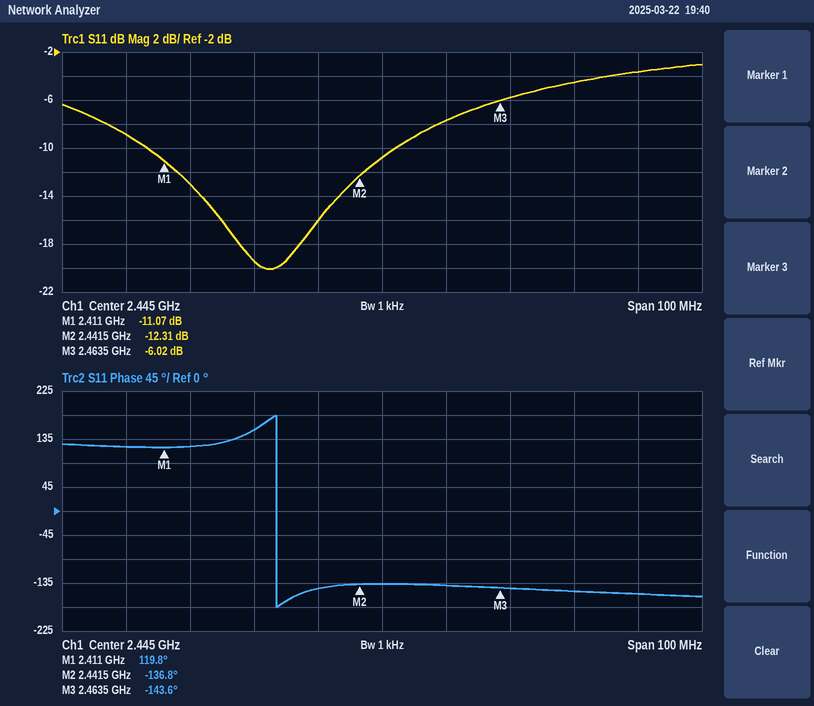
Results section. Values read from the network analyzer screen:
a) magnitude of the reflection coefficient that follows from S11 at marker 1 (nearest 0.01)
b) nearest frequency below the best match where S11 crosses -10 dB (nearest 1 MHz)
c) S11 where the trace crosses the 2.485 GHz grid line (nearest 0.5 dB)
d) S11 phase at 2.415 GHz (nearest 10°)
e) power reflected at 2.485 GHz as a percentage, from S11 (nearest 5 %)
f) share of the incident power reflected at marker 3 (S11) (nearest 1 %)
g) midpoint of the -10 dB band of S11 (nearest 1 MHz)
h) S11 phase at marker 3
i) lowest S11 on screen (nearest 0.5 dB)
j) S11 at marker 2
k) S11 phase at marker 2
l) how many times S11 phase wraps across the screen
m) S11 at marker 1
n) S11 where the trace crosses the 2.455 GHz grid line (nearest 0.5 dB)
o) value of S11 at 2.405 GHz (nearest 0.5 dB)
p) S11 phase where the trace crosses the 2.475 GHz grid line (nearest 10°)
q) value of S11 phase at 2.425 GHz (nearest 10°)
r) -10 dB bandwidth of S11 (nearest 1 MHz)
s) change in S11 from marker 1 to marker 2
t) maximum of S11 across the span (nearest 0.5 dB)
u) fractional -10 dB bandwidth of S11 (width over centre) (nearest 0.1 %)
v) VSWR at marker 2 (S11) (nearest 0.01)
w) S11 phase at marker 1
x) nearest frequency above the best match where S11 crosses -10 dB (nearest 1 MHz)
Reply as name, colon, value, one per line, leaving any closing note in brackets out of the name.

magnitude of the reflection coefficient that follows from S11 at marker 1: 0.28
nearest frequency below the best match where S11 crosses -10 dB: 2.408 GHz
S11 where the trace crosses the 2.485 GHz grid line: -3.5 dB
S11 phase at 2.415 GHz: 120°
power reflected at 2.485 GHz as a percentage, from S11: 45 %
share of the incident power reflected at marker 3 (S11): 25 %
midpoint of the -10 dB band of S11: 2.428 GHz
S11 phase at marker 3: -143.6°
lowest S11 on screen: -20.0 dB
S11 at marker 2: -12.31 dB
S11 phase at marker 2: -136.8°
how many times S11 phase wraps across the screen: 1
S11 at marker 1: -11.07 dB
S11 where the trace crosses the 2.455 GHz grid line: -7.5 dB
value of S11 at 2.405 GHz: -9.0 dB
S11 phase where the trace crosses the 2.475 GHz grid line: -150°
value of S11 phase at 2.425 GHz: 150°
-10 dB bandwidth of S11: 39 MHz
change in S11 from marker 1 to marker 2: -1.24 dB
maximum of S11 across the span: -3.0 dB
fractional -10 dB bandwidth of S11 (width over centre): 1.6 %
VSWR at marker 2 (S11): 1.64
S11 phase at marker 1: 119.8°
nearest frequency above the best match where S11 crosses -10 dB: 2.447 GHz
